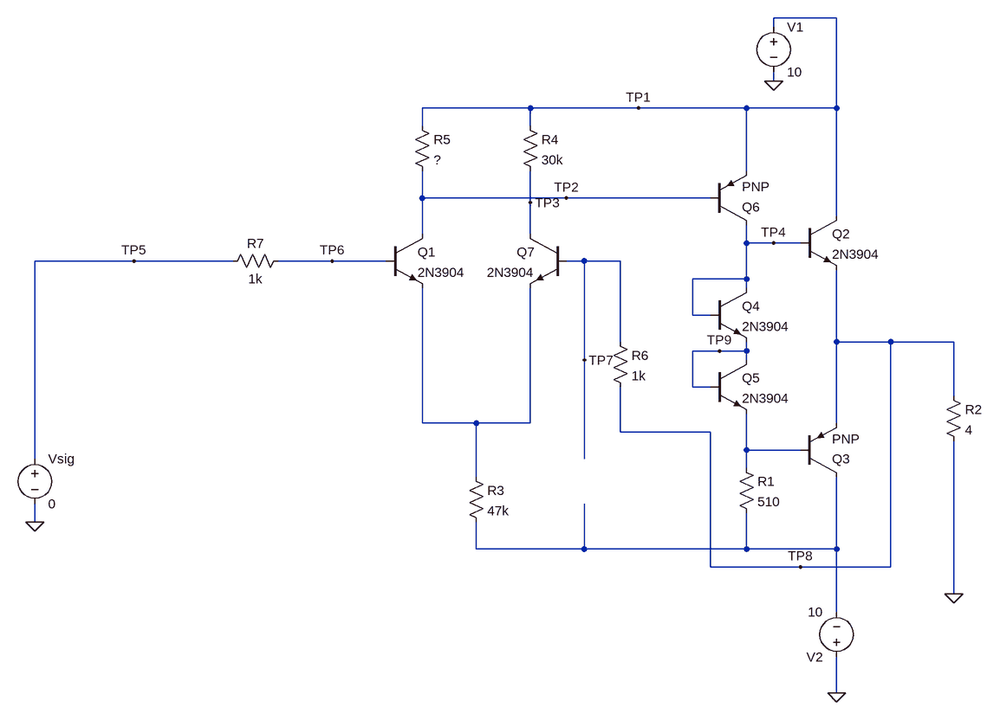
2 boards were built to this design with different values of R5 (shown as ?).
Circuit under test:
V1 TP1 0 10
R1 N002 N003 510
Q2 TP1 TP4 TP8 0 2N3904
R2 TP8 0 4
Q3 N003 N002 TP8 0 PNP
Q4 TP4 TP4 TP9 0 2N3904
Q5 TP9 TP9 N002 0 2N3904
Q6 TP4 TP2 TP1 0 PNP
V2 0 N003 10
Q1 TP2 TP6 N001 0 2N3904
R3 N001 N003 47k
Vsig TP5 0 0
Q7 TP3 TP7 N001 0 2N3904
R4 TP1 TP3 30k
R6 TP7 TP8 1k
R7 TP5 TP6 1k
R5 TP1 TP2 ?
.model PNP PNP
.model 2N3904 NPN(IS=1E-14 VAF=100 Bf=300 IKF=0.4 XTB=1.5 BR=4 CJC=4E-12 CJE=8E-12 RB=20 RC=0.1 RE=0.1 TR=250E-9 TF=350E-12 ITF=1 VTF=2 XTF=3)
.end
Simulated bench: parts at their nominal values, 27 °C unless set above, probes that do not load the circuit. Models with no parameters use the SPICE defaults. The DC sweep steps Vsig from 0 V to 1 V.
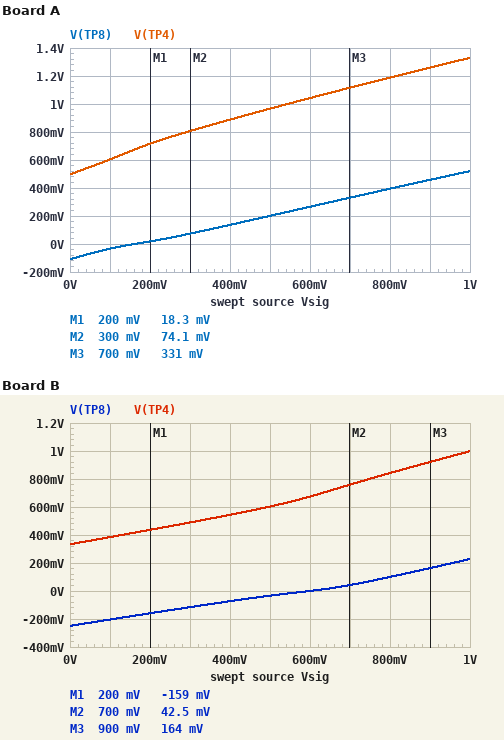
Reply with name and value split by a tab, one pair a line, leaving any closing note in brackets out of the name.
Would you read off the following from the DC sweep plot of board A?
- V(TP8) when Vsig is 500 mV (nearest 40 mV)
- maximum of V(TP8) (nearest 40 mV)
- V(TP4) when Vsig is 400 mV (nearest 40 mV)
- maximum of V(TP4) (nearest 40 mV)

V(TP8) when Vsig is 500 mV	200 mV
maximum of V(TP8)	520 mV
V(TP4) when Vsig is 400 mV	880 mV
maximum of V(TP4)	1.32 V
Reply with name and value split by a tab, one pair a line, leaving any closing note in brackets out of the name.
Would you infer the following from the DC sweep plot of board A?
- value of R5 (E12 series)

value of R5	39 kΩ
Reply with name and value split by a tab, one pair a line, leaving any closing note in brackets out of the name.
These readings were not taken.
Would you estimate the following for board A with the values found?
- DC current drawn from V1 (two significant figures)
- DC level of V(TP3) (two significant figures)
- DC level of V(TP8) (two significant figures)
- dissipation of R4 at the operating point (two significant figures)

DC current drawn from V1	18 mA
DC level of V(TP3)	9.9 V
DC level of V(TP8)	-110 mV
dissipation of R4 at the operating point	270 nW
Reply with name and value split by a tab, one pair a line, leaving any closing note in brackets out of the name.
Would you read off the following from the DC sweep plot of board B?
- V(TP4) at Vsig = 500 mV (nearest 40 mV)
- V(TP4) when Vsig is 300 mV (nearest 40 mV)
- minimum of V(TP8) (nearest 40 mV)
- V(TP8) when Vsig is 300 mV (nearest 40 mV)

V(TP4) at Vsig = 500 mV	600 mV
V(TP4) when Vsig is 300 mV	480 mV
minimum of V(TP8)	-240 mV
V(TP8) when Vsig is 300 mV	-120 mV
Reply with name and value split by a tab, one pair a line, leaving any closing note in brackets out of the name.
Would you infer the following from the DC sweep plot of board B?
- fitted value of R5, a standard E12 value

fitted value of R5, a standard E12 value	27 kΩ
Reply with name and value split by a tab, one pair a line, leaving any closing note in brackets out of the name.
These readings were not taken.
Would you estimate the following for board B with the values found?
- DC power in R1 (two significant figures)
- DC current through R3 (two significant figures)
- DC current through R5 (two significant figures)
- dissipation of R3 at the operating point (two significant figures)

DC power in R1	150 mW
DC current through R3	200 µA
DC current through R5	31 µA
dissipation of R3 at the operating point	1.9 mW
